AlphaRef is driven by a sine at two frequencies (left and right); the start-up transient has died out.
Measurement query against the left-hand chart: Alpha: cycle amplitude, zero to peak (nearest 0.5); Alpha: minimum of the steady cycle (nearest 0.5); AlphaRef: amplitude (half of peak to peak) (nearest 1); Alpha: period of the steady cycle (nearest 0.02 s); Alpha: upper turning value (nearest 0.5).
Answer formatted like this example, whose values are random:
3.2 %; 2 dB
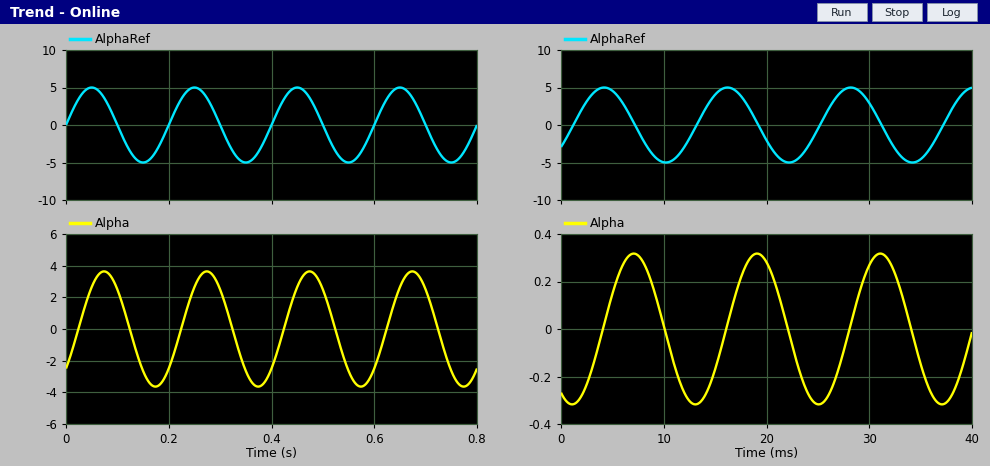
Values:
3.5; -3.5; 5; 0.20 s; 3.5
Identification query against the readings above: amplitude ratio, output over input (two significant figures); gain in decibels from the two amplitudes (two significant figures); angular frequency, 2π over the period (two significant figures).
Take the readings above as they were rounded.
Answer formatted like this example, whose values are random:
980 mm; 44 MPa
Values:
0.70; -3.1 dB; 31 rad/s
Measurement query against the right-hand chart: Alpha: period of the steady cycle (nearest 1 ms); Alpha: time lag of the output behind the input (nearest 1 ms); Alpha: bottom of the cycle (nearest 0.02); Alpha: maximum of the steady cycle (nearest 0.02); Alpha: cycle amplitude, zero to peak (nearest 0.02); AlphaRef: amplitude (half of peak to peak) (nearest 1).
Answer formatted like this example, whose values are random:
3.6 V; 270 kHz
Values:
12 ms; 3 ms; -0.32; 0.32; 0.32; 5
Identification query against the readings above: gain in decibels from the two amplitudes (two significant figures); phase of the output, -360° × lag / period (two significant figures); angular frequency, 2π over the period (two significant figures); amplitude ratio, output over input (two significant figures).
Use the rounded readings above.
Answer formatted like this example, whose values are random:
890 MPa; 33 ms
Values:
-24 dB; -90°; 0.52 rad/ms; 0.064
